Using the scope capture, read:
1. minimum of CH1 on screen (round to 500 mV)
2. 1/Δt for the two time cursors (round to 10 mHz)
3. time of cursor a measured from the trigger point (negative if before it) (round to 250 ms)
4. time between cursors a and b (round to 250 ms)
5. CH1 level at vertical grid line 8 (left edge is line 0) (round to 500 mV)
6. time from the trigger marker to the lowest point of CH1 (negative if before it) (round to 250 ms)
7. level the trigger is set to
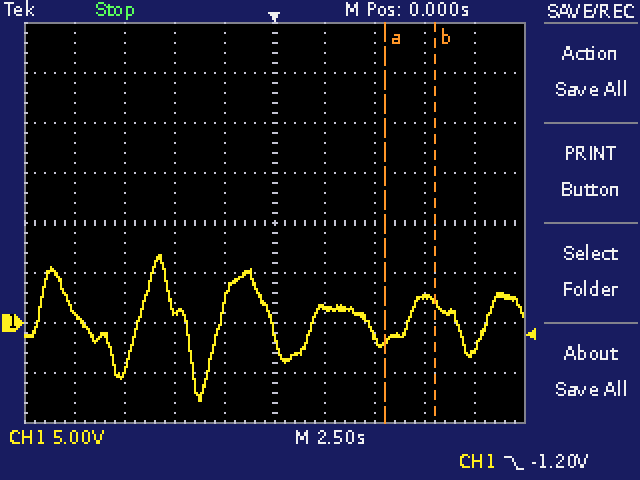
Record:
-8.0 V
400 mHz
+5.50 s
2.50 s
2.5 V
-3.75 s
-1.20 V
